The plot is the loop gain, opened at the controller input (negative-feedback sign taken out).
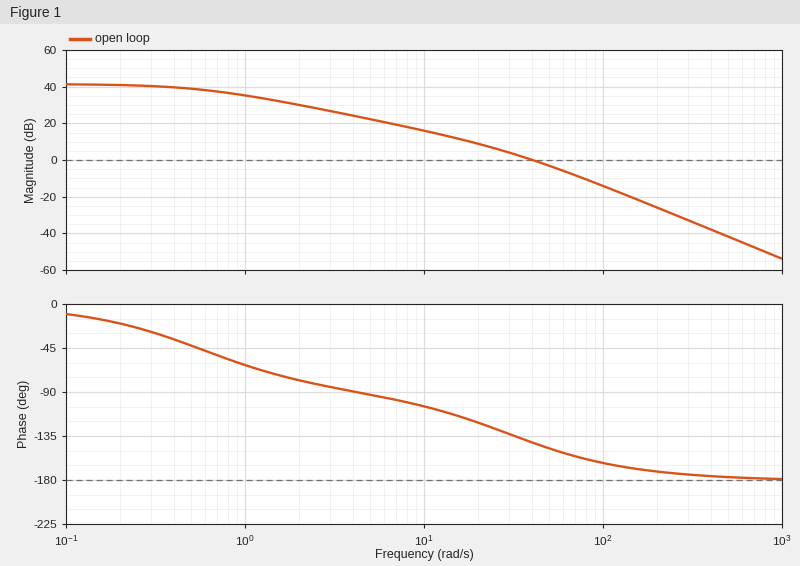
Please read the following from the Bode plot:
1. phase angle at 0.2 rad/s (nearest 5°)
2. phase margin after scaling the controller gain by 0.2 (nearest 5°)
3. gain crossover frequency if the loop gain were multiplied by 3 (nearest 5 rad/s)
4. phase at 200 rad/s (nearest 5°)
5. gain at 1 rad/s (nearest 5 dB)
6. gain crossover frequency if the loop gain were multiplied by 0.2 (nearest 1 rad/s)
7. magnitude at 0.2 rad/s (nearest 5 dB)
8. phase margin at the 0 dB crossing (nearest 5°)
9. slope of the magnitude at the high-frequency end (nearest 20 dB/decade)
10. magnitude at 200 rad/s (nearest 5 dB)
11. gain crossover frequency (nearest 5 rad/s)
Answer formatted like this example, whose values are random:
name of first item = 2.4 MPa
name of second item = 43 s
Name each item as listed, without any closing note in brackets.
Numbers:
phase angle at 0.2 rad/s = -20°
phase margin after scaling the controller gain by 0.2 = 70°
gain crossover frequency if the loop gain were multiplied by 3 = 75 rad/s
phase at 200 rad/s = -170°
gain at 1 rad/s = 35 dB
gain crossover frequency if the loop gain were multiplied by 0.2 = 12 rad/s
magnitude at 0.2 rad/s = 40 dB
phase margin at the 0 dB crossing = 40°
slope of the magnitude at the high-frequency end = -40 dB/decade
magnitude at 200 rad/s = -25 dB
gain crossover frequency = 40 rad/s
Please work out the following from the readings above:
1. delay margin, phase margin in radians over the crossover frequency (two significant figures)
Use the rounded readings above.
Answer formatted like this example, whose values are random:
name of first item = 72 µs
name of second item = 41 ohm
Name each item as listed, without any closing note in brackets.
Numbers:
delay margin, phase margin in radians over the crossover frequency = 0.017 s
